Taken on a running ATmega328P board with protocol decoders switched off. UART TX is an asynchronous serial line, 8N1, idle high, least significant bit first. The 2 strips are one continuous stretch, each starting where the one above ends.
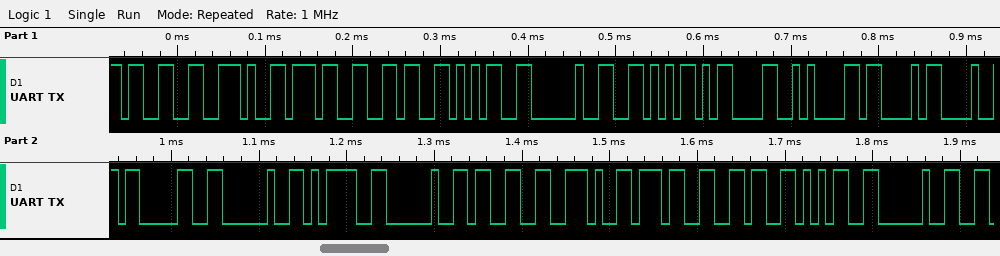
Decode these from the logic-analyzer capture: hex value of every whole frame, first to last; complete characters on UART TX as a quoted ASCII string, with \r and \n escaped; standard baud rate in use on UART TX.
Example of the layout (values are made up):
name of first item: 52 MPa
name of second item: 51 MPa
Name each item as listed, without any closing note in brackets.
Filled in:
hex value of every whole frame, first to last: 33 2E 37 36 35 20 56 0D 0A 43 48 30 20 3D 20 33 2E 37 36 35 20
complete characters on UART TX as a quoted ASCII string, with \r and \n escaped: "3.765 V\r\nCH0 = 3.765 "
standard baud rate in use on UART TX: 115200 baud
